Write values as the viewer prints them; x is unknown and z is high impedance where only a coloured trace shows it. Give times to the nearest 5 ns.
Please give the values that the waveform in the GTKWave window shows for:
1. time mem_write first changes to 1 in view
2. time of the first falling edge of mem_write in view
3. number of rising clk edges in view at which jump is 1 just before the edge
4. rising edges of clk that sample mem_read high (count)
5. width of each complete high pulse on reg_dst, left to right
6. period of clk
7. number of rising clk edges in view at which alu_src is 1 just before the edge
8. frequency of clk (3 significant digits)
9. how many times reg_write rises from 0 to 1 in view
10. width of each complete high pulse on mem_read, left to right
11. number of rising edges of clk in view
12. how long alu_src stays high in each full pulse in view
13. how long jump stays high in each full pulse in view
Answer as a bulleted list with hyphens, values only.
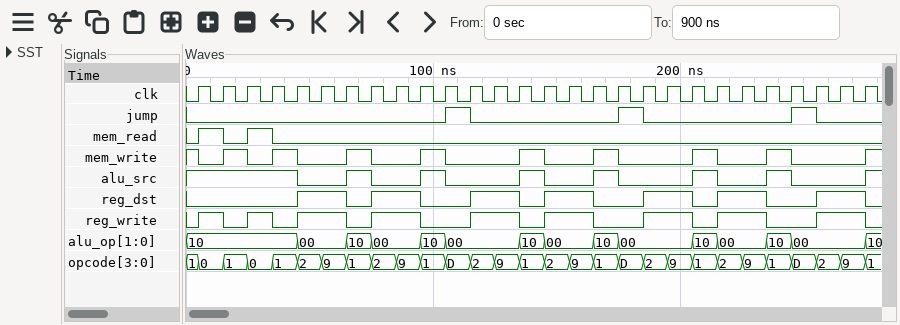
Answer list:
- 15 ns
- 5 ns
- 3
- 2
- 20 ns, 20 ns, 20 ns, 20 ns, 20 ns, 20 ns, 20 ns
- 10 ns
- 11
- 100 MHz
- 9
- 10 ns, 10 ns
- 28
- 10 ns, 10 ns, 10 ns, 10 ns, 10 ns, 10 ns
- 10 ns, 10 ns, 10 ns
